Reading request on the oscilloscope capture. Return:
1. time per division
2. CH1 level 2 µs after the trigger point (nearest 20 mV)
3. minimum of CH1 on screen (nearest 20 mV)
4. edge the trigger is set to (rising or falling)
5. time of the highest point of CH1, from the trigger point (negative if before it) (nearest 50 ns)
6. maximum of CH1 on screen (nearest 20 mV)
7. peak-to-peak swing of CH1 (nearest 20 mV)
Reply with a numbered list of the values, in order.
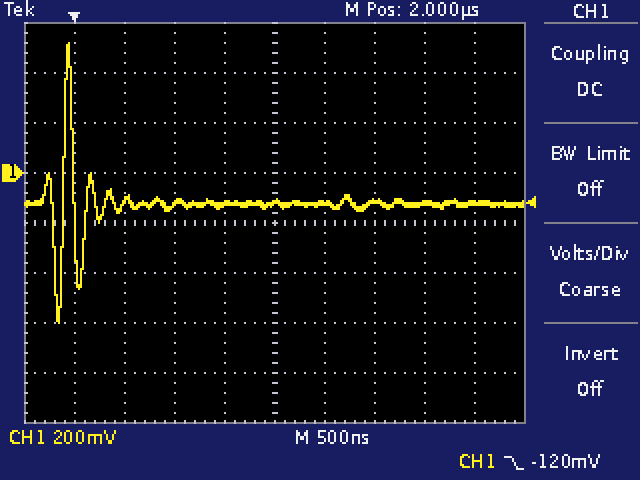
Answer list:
1. 500 ns
2. -120 mV
3. -600 mV
4. falling
5. -50 ns
6. 520 mV
7. 1.12 V
